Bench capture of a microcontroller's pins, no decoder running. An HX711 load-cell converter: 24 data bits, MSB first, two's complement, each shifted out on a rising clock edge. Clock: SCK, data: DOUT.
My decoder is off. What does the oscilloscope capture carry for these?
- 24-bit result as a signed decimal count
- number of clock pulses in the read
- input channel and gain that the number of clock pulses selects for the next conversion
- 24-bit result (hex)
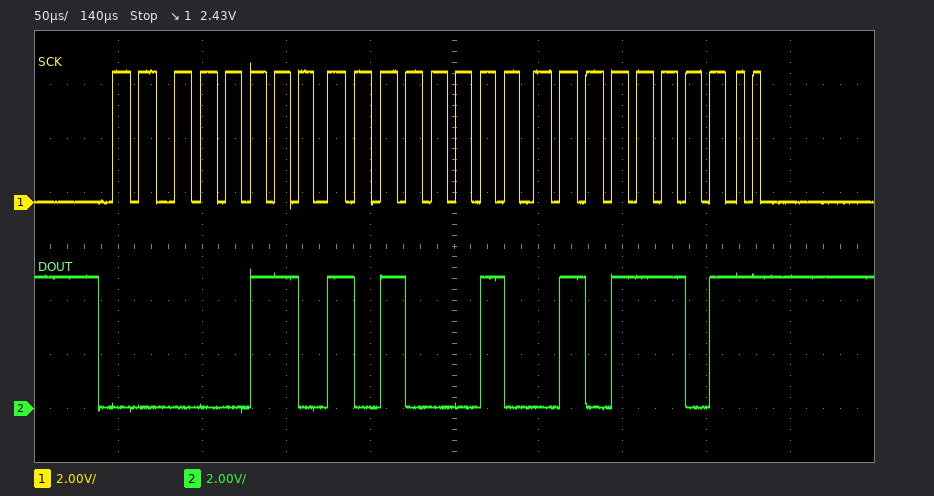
434781
26
channel B, gain 32
0x06A25D
